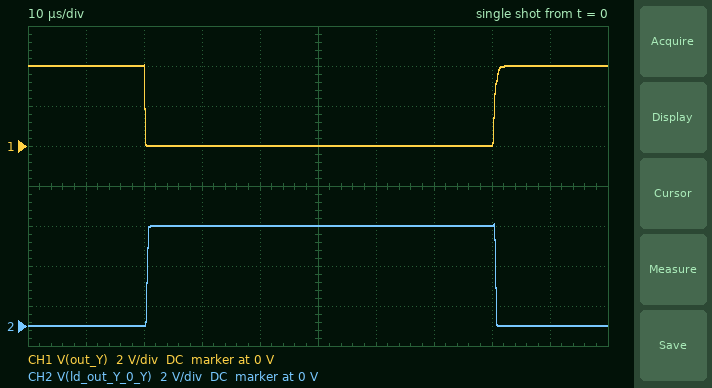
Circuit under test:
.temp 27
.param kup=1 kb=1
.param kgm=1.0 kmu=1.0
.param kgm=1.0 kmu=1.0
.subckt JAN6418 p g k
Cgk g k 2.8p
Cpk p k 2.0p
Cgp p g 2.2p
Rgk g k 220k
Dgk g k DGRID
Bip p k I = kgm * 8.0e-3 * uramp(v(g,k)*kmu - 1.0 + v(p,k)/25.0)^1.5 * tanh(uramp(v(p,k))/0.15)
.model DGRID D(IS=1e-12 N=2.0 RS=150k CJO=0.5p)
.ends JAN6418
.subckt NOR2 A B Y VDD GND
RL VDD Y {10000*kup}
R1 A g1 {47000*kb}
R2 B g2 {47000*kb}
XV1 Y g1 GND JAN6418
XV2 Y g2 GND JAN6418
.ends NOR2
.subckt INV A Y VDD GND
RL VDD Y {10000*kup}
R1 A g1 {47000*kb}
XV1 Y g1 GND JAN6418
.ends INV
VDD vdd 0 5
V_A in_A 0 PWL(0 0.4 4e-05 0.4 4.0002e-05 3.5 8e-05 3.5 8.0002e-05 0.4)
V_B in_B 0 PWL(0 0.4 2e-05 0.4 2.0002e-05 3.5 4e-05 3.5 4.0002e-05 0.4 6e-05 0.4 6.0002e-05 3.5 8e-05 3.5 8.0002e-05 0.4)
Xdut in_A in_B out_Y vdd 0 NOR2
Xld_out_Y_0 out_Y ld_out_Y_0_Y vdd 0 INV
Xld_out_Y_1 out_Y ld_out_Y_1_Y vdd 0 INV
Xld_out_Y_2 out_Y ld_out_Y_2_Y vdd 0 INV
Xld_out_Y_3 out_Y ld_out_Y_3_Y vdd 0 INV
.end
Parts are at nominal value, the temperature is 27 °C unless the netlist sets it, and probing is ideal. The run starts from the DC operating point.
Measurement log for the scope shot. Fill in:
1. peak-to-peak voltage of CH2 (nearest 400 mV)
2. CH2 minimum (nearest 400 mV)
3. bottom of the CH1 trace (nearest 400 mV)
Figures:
5.2 V
0 V
0 V
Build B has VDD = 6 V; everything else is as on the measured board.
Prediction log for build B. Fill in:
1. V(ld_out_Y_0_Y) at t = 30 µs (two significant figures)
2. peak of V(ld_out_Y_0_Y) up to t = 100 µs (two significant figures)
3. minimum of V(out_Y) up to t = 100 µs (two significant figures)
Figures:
6.0 V
6.1 V
2.9 mV
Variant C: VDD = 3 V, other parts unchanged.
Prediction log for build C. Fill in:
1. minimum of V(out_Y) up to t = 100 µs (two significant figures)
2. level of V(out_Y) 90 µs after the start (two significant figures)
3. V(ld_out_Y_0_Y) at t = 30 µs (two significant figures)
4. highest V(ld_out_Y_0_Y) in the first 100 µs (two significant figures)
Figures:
1.3 mV
2.4 V
3.0 V
3.1 V
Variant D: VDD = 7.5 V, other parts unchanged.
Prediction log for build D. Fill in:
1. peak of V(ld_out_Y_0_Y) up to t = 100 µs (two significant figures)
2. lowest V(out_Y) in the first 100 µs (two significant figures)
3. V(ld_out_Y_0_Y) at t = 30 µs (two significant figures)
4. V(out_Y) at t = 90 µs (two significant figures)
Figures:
7.6 V
3.7 mV
7.5 V
5.9 V
